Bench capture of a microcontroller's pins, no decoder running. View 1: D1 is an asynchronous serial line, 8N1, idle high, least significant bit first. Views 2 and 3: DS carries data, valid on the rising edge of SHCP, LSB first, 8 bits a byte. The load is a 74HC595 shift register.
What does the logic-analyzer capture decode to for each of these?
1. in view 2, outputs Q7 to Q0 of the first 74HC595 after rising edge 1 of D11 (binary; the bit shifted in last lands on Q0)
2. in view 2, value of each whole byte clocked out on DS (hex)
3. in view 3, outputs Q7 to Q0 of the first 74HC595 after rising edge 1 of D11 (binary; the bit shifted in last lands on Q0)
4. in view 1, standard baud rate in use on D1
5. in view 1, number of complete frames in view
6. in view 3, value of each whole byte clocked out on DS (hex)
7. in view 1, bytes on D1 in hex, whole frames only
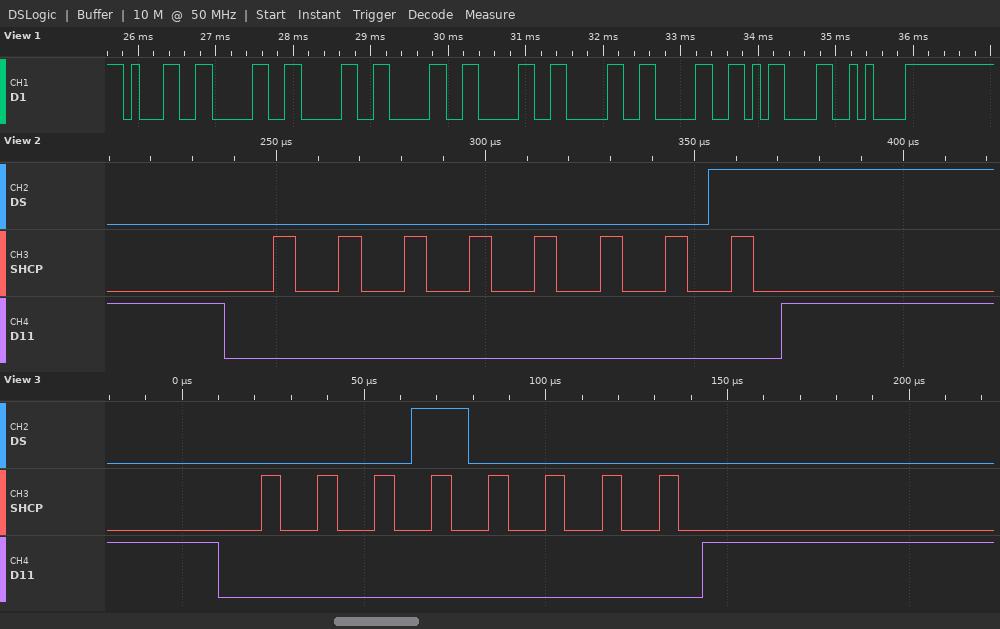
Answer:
00000001
80
00010000
9600 baud
9
08
31 30 30 30 30 30 30 0D 0A
